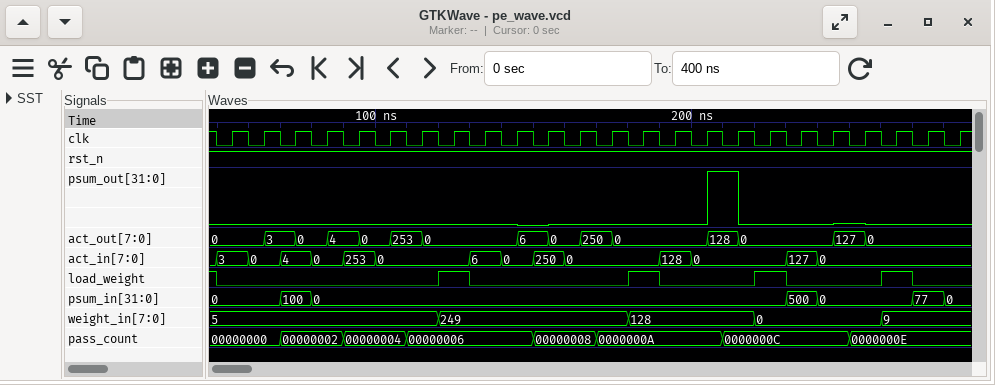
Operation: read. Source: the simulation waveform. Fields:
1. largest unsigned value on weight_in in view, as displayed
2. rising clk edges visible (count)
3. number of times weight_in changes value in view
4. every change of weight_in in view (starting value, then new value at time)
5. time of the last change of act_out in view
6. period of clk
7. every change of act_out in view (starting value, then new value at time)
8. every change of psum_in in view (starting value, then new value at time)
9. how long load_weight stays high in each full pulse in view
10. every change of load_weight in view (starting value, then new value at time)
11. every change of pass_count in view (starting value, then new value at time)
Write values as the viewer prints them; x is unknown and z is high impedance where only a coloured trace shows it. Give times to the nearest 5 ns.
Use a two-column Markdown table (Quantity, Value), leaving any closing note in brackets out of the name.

| Quantity | Value |
|---|---|
| largest unsigned value on weight_in in view, as displayed | 249 |
| rising clk edges visible | 24 |
| number of times weight_in changes value in view | 4 |
| every change of weight_in in view | 5, 249 at 120 ns, 128 at 180 ns, 0 at 220 ns, 9 at 260 ns |
| time of the last change of act_out in view | 255 ns |
| period of clk | 10 ns |
| every change of act_out in view | 0, 3 at 65 ns, 0 at 75 ns, 4 at 85 ns, 0 at 95 ns, 253 at 105 ns, 0 at 115 ns, 6 at 145 ns, 0 at 155 ns, 250 at 165 ns, 0 at 175 ns, 128 at 205 ns, 0 at 215 ns, 127 at 245 ns, 0 at 255 ns |
| every change of psum_in in view | 0, 100 at 70 ns, 0 at 80 ns, 500 at 230 ns, 0 at 240 ns, 77 at 270 ns, 0 at 280 ns |
| how long load_weight stays high in each full pulse in view | 10 ns, 10 ns, 10 ns, 10 ns |
| every change of load_weight in view | 1, 0 at 50 ns, 1 at 120 ns, 0 at 130 ns, 1 at 180 ns, 0 at 190 ns, 1 at 220 ns, 0 at 230 ns, 1 at 260 ns, 0 at 270 ns |
| every change of pass_count in view | 00000000, 00000002 at 70 ns, 00000004 at 90 ns, 00000006 at 110 ns, 00000008 at 150 ns, 0000000A at 170 ns, 0000000C at 210 ns, 0000000E at 250 ns |
